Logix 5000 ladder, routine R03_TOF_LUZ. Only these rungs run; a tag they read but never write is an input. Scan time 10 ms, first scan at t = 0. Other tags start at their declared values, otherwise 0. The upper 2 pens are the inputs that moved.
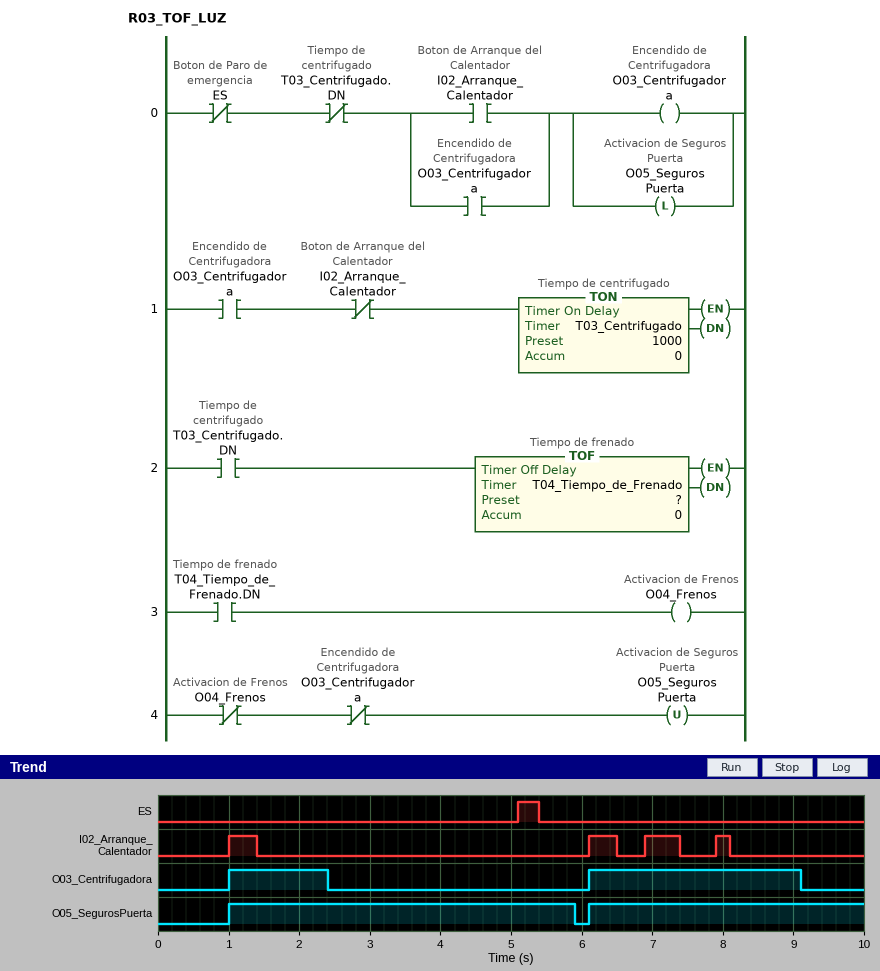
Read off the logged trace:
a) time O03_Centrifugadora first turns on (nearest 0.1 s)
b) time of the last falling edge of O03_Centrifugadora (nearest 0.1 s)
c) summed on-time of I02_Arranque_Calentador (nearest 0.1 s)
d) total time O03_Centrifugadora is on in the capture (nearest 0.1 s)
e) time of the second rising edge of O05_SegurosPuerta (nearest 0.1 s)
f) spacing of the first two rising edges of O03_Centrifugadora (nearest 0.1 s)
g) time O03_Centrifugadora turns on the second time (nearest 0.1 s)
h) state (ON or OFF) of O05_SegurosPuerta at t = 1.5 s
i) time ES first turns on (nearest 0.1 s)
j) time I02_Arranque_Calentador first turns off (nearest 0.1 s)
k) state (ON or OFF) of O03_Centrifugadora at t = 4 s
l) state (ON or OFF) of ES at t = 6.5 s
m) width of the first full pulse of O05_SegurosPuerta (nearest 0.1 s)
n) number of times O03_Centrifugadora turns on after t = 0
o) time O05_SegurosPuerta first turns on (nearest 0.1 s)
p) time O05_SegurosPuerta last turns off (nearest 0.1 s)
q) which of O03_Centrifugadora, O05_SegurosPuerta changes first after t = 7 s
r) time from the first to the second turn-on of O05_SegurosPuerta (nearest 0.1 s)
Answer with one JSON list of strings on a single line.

["1.0 s", "9.1 s", "1.5 s", "4.4 s", "6.1 s", "5.1 s", "6.1 s", "ON", "5.1 s", "1.4 s", "OFF", "OFF", "4.9 s", "2", "1.0 s", "5.9 s", "O03_Centrifugadora", "5.1 s"]
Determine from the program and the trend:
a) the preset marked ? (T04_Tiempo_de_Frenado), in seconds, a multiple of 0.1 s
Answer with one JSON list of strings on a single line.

["3.5 s"]
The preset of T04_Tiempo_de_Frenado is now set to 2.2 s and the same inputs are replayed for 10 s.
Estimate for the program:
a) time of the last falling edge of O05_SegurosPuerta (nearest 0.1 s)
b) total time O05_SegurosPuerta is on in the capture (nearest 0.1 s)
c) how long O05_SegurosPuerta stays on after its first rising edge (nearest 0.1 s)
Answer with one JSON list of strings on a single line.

["4.6 s", "7.5 s", "3.6 s"]
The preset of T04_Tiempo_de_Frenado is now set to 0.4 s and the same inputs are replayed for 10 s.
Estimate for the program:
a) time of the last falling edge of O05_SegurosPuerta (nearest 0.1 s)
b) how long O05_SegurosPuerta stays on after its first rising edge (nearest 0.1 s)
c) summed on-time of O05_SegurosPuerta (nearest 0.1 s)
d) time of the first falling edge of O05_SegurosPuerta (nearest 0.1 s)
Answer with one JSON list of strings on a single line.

["9.5 s", "1.8 s", "5.2 s", "2.8 s"]
